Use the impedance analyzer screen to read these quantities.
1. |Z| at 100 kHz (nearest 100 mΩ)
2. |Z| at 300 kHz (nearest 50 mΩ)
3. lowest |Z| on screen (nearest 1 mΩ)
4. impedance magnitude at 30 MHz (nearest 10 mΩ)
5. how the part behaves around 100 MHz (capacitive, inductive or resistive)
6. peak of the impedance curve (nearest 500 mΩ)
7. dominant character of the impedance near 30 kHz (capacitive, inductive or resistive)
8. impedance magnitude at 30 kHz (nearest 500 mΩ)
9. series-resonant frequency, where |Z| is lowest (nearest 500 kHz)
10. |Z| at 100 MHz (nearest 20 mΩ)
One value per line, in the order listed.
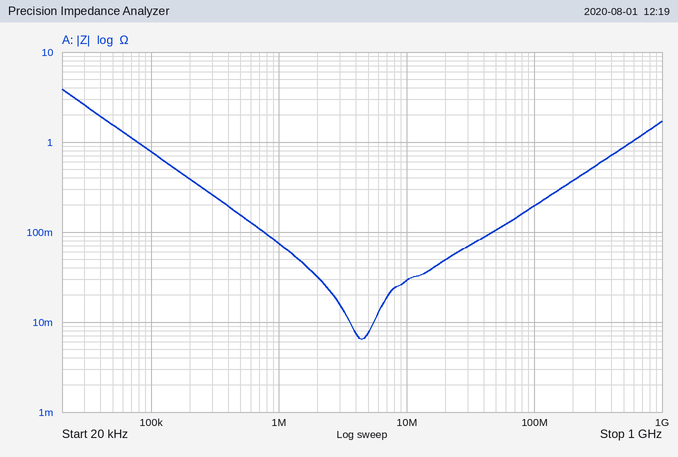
800 mΩ
250 mΩ
6 mΩ
70 mΩ
inductive
4.0 Ω
capacitive
2.5 Ω
4.5 MHz
200 mΩ
